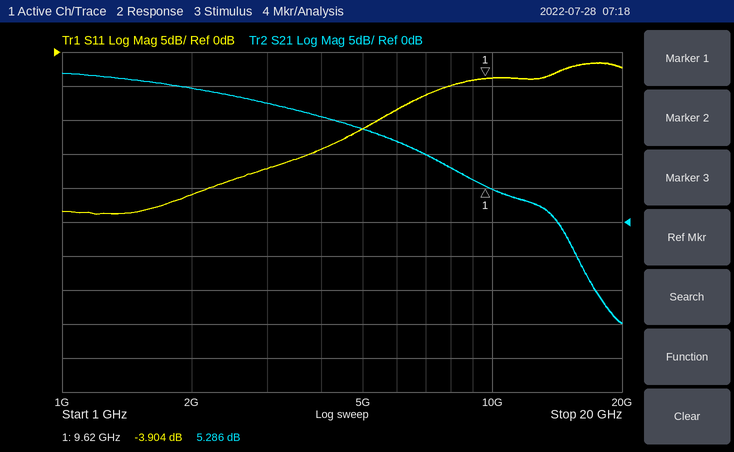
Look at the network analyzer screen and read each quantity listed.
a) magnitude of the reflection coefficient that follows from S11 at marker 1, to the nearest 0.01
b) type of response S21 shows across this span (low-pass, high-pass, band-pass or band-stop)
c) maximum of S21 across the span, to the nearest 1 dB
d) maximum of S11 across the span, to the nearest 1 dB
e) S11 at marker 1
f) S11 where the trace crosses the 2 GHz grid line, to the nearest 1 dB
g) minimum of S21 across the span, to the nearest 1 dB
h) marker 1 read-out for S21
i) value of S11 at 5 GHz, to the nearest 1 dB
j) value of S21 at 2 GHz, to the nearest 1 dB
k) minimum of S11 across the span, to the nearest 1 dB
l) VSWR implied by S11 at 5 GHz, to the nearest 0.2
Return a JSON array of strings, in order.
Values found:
["0.64", "low-pass", "22 dB", "-2 dB", "-3.904 dB", "-21 dB", "-15 dB", "5.286 dB", "-11 dB", "20 dB", "-24 dB", "1.8"]
